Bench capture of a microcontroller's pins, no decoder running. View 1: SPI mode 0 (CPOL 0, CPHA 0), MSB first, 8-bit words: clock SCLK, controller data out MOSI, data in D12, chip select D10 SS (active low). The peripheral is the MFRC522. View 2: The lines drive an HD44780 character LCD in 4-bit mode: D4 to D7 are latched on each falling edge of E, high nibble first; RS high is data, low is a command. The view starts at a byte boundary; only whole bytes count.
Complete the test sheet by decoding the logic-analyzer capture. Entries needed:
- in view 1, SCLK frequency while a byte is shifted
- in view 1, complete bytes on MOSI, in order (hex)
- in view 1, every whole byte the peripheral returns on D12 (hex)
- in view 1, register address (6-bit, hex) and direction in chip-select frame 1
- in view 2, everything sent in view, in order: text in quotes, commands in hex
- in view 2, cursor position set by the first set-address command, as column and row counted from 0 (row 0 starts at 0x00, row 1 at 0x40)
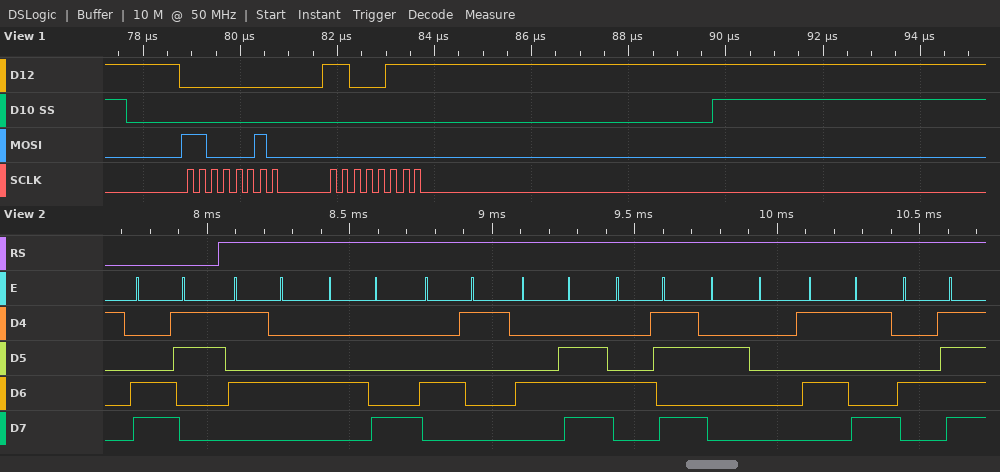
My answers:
4 MHz
C2 00
00 C7
0x21 read
0xC3 "THANK YO"
column 3, row 1
